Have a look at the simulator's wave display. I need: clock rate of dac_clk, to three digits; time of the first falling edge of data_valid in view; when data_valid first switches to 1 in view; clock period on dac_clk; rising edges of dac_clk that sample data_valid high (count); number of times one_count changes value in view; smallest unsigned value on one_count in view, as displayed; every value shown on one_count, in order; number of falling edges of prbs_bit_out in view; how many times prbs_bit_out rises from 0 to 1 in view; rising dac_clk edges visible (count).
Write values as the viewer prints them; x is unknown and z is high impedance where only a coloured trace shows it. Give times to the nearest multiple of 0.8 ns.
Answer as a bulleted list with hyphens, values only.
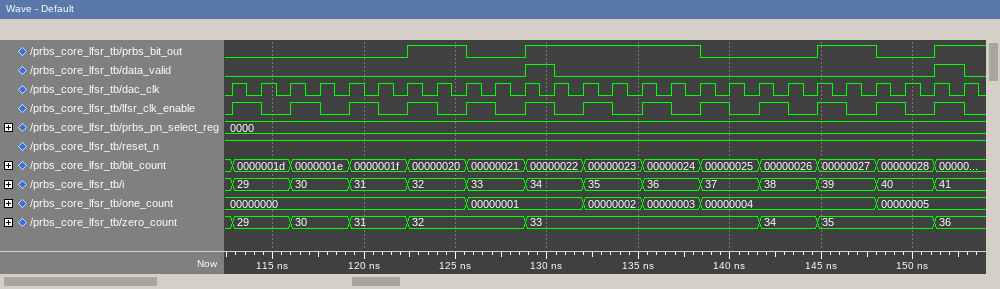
- 625 MHz
- 130.4 ns
- 128.8 ns
- 1.6 ns
- 2
- 5
- 00000000
- 00000000, 00000001, 00000002, 00000003, 00000004, 00000005
- 3
- 4
- 26
